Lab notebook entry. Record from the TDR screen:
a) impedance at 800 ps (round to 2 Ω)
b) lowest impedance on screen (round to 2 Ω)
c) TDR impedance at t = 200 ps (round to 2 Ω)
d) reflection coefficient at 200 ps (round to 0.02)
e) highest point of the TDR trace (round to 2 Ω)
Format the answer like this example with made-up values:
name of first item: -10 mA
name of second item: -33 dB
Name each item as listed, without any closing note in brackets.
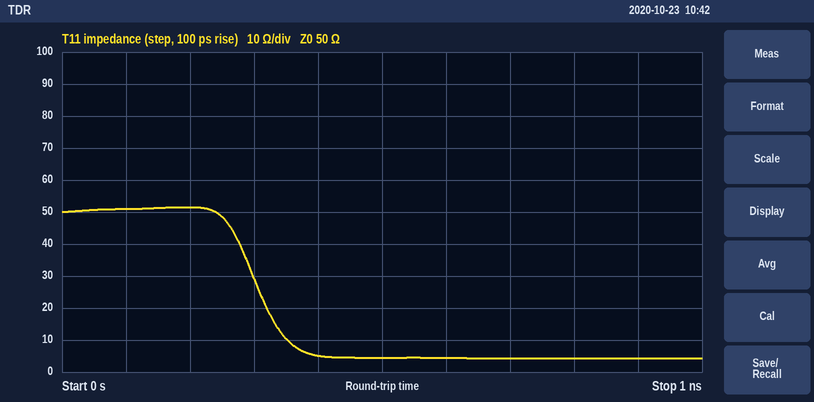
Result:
impedance at 800 ps: 4 Ω
lowest impedance on screen: 4 Ω
TDR impedance at t = 200 ps: 52 Ω
reflection coefficient at 200 ps: +0.02
highest point of the TDR trace: 52 Ω
